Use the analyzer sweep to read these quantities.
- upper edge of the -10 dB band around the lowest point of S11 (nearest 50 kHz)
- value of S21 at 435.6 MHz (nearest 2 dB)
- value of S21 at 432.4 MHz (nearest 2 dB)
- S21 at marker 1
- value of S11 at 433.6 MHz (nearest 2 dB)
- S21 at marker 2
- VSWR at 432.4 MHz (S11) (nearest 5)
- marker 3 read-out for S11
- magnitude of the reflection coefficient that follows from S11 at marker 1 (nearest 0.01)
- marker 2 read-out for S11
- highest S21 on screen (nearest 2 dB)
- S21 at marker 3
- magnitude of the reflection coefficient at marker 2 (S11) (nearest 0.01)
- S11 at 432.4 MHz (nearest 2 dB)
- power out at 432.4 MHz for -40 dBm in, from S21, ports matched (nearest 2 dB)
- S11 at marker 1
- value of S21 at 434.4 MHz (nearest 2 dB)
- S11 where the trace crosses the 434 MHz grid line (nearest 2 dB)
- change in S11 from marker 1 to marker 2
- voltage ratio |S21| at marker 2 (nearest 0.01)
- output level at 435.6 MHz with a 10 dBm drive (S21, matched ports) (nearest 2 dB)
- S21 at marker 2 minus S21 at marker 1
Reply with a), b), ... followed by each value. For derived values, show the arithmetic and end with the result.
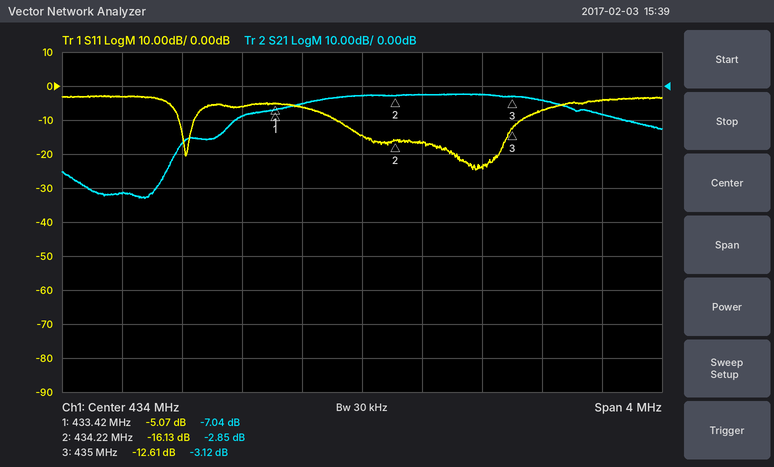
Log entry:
a) 435.05 MHz
b) -8 dB
c) -32 dB
d) -7.04 dB
e) -6 dB
f) -2.85 dB
g) |Γ| = 10^(-4/20) = 0.6310; VSWR = (1 + 0.6310)/(1 − 0.6310) ≈ 4.42, so 5 to the nearest 5
h) -12.61 dB
i) 10^(-5.07/20) ≈ 0.56
j) -16.13 dB
k) -2 dB
l) -3.12 dB
m) 10^(-16.13/20) ≈ 0.16
n) -4 dB
o) -40 dBm + (-32 dB) = -72 dBm
p) -5.07 dB
q) -2 dB
r) -14 dB
s) -16.13 − (-5.07) = -11.06 dB
t) 10^(-2.85/20) ≈ 0.72
u) 10 dBm + (-8 dB) = 2 dBm
v) -2.85 − (-7.04) = 4.19 dB
